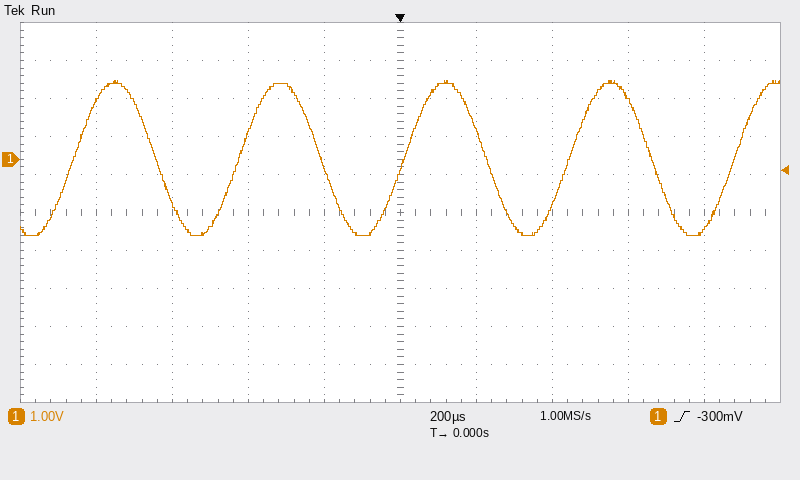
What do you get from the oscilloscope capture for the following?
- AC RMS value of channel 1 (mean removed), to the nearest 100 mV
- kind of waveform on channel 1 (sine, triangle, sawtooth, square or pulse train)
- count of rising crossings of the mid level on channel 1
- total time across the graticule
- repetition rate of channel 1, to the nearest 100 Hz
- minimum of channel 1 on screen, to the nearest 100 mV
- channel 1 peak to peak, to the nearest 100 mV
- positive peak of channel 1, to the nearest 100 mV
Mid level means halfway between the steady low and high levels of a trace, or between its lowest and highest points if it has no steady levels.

1.4 V
sine
5
2 ms
2.3 kHz
-2.0 V
4.1 V
2.1 V
